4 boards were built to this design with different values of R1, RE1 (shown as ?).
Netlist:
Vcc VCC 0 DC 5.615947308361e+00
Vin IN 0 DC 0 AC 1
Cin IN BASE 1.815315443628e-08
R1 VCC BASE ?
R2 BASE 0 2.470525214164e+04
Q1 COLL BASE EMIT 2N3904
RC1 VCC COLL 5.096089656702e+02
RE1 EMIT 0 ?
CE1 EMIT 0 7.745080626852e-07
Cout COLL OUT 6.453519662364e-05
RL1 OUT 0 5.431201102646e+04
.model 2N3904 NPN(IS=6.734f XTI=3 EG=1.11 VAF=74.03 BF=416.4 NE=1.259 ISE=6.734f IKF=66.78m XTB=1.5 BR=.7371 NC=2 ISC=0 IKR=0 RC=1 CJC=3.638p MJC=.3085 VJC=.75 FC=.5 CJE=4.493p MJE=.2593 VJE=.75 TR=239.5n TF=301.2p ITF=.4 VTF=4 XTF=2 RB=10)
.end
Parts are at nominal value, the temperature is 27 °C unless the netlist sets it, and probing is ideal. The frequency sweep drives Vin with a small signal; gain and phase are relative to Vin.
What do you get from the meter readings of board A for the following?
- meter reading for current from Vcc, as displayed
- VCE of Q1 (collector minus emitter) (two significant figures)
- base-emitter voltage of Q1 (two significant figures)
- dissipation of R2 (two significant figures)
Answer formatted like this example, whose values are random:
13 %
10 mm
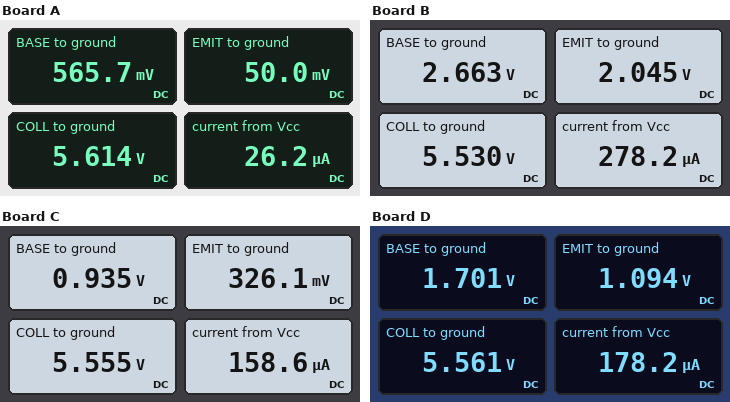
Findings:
26.2 µA
5.6 V
520 mV
13 µW
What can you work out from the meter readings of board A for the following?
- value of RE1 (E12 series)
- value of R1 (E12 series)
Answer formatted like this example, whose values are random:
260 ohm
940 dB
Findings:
15 kΩ
220 kΩ
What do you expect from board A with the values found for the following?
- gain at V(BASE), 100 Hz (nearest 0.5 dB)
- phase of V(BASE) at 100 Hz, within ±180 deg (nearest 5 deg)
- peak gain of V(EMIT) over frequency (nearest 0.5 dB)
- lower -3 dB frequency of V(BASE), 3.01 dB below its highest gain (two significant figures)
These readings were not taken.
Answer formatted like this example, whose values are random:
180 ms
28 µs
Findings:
-12.5 dB
75 deg
-24.5 dB
410 Hz
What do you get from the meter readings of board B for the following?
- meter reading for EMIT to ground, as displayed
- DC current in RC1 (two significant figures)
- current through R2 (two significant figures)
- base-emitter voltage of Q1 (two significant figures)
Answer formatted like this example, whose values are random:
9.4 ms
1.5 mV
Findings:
2.045 V
170 µA
110 µA
620 mV
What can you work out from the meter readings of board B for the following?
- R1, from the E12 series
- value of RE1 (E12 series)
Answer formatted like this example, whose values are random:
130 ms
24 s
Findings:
27 kΩ
12 kΩ
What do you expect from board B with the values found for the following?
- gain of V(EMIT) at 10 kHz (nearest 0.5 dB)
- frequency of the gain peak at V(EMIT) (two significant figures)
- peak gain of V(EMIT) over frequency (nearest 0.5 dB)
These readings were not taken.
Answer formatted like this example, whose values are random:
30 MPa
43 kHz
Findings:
-17.5 dB
970 Hz
-5.5 dB
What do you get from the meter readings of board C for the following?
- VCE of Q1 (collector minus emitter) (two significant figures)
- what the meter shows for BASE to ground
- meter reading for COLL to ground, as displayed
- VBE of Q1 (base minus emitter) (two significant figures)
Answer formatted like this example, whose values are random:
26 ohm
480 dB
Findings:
5.2 V
0.935 V
5.555 V
610 mV
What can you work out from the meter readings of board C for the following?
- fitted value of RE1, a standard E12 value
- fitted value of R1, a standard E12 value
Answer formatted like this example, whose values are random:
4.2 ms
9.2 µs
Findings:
2.7 kΩ
120 kΩ
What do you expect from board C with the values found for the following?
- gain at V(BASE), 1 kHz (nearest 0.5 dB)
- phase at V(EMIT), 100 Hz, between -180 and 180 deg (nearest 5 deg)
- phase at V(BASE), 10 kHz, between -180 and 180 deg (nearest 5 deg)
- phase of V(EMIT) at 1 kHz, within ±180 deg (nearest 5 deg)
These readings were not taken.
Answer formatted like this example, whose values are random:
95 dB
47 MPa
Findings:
-2.5 dB
70 deg
5 deg
-15 deg
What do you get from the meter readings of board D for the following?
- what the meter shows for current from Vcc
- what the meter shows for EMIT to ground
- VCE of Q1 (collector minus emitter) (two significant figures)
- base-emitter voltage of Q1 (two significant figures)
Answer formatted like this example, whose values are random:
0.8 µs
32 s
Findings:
178.2 µA
1.094 V
4.5 V
610 mV
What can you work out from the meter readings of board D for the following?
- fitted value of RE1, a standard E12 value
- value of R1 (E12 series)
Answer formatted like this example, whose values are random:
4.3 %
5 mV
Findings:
10 kΩ
56 kΩ
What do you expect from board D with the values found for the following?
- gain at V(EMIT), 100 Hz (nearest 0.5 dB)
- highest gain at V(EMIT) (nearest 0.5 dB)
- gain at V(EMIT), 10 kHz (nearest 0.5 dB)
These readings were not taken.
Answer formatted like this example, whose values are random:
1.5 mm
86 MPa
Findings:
-15.0 dB
-6.0 dB
-21.5 dB
